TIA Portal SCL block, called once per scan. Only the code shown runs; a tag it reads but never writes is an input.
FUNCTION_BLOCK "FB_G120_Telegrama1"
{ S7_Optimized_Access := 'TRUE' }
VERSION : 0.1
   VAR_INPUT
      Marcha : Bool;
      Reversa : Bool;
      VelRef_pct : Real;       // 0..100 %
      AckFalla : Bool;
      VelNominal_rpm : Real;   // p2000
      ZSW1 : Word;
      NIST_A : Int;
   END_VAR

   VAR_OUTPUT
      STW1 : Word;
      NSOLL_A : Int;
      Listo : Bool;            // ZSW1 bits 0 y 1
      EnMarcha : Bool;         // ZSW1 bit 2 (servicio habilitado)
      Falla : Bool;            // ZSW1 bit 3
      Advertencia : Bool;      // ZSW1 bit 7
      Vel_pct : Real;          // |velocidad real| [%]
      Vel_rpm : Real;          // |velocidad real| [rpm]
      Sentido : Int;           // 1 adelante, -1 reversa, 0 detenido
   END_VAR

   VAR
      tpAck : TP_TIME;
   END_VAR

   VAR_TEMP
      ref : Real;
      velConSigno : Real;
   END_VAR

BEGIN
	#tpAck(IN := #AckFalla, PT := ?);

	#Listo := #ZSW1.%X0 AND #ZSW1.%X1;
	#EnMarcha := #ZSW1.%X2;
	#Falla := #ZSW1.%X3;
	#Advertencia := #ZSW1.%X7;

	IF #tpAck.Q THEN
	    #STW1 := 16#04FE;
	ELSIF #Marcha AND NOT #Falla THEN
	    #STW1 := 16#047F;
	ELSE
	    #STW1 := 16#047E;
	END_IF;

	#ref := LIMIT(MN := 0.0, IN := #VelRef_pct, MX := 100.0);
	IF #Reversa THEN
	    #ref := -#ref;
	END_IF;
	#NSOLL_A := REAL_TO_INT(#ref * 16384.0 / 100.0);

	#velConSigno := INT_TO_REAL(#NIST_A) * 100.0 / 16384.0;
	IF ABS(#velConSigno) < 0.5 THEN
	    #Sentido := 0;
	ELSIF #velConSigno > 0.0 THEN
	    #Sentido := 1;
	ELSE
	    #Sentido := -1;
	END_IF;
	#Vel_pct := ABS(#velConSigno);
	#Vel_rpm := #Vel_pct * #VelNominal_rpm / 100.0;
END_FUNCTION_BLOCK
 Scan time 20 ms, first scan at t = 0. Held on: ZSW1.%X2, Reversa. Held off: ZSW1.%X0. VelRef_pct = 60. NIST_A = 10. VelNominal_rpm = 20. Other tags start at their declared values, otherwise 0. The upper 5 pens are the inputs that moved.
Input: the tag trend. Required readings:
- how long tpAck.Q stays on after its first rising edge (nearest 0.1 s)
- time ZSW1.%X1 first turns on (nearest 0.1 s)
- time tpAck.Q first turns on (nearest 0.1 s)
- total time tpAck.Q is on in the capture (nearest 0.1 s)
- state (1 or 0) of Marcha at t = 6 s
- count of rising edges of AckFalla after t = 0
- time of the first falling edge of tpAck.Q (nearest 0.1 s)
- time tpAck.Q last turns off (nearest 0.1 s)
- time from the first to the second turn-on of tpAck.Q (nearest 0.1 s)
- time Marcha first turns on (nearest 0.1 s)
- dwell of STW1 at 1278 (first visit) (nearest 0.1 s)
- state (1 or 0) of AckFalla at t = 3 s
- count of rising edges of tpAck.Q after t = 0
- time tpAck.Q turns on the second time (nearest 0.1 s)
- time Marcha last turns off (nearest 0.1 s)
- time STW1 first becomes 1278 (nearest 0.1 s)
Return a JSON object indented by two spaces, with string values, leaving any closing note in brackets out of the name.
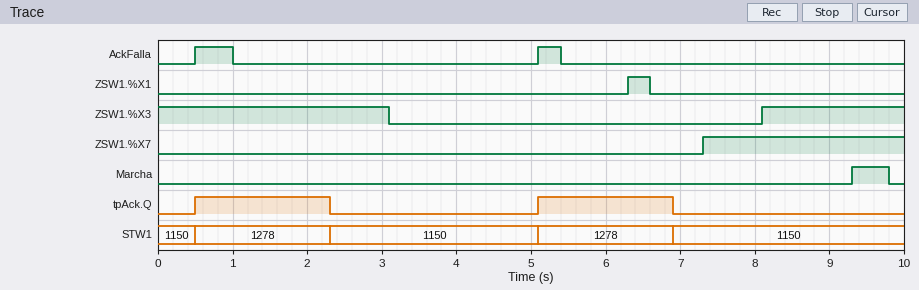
{
  "how long tpAck.Q stays on after its first rising edge": "1.8 s",
  "time ZSW1.%X1 first turns on": "6.3 s",
  "time tpAck.Q first turns on": "0.5 s",
  "total time tpAck.Q is on in the capture": "3.6 s",
  "state (1 or 0) of Marcha at t = 6 s": "0",
  "count of rising edges of AckFalla after t = 0": "2",
  "time of the first falling edge of tpAck.Q": "2.3 s",
  "time tpAck.Q last turns off": "6.9 s",
  "time from the first to the second turn-on of tpAck.Q": "4.6 s",
  "time Marcha first turns on": "9.3 s",
  "dwell of STW1 at 1278 (first visit)": "1.8 s",
  "state (1 or 0) of AckFalla at t = 3 s": "0",
  "count of rising edges of tpAck.Q after t = 0": "2",
  "time tpAck.Q turns on the second time": "5.1 s",
  "time Marcha last turns off": "9.8 s",
  "time STW1 first becomes 1278": "0.5 s"
}
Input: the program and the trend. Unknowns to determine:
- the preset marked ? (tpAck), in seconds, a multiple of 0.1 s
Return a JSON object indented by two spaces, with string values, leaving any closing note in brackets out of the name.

{
  "the preset marked ? (tpAck), in seconds, a multiple of 0.1 s": "1.8 s"
}
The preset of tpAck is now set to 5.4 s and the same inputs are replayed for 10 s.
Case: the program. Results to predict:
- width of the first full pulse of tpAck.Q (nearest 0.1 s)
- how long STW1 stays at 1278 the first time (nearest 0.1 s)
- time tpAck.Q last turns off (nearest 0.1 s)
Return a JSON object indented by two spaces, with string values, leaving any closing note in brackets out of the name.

{
  "width of the first full pulse of tpAck.Q": "5.4 s",
  "how long STW1 stays at 1278 the first time": "5.4 s",
  "time tpAck.Q last turns off": "5.9 s"
}
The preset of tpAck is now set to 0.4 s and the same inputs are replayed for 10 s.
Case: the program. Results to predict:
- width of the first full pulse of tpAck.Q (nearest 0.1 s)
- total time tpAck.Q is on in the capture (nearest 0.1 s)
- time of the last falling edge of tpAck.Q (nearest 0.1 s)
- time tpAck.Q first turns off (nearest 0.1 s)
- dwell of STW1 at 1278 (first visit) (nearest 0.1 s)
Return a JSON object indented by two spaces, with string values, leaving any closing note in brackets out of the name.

{
  "width of the first full pulse of tpAck.Q": "0.4 s",
  "total time tpAck.Q is on in the capture": "0.8 s",
  "time of the last falling edge of tpAck.Q": "5.5 s",
  "time tpAck.Q first turns off": "0.9 s",
  "dwell of STW1 at 1278 (first visit)": "0.4 s"
}
